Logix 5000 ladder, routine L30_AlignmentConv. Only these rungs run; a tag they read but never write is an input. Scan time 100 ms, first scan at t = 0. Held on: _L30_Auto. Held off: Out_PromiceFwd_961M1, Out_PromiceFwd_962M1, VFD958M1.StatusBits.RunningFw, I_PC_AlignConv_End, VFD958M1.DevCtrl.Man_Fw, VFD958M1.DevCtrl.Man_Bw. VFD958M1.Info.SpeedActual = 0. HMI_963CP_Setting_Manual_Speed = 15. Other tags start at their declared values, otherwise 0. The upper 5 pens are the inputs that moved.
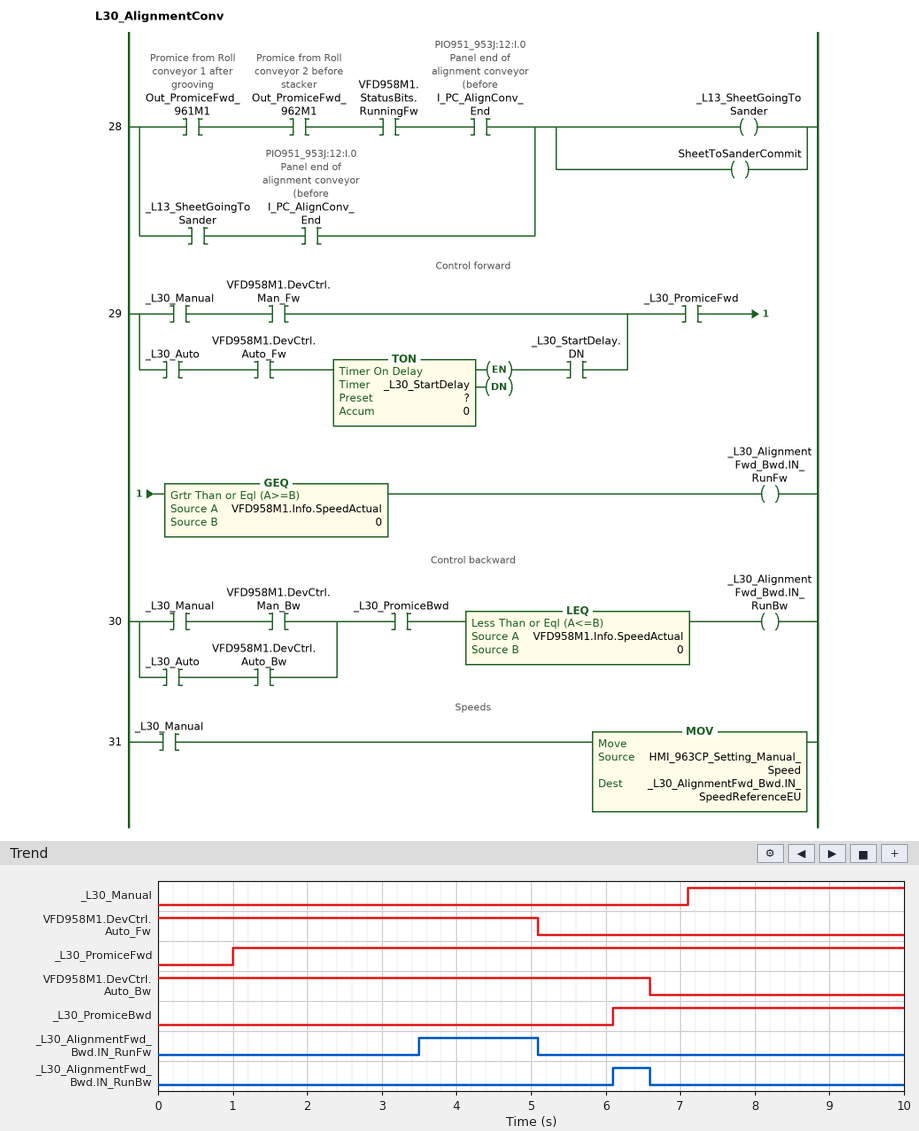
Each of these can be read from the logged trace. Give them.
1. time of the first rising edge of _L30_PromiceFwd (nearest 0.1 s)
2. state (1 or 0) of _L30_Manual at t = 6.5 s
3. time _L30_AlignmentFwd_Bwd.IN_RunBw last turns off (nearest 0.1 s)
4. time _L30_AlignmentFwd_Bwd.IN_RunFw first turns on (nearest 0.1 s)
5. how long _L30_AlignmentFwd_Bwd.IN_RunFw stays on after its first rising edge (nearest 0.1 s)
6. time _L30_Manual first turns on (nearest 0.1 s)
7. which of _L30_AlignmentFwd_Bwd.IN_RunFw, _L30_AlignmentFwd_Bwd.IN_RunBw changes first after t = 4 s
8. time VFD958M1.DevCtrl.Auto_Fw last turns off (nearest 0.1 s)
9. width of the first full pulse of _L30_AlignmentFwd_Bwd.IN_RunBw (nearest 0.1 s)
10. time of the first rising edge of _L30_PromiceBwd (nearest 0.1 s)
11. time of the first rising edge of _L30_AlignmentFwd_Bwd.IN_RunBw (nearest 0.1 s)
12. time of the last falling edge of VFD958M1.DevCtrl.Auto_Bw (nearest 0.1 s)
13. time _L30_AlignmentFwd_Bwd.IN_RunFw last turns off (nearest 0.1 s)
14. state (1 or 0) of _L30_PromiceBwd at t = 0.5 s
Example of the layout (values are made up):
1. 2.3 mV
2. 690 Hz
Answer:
1. 1.0 s
2. 0
3. 6.6 s
4. 3.5 s
5. 1.6 s
6. 7.1 s
7. _L30_AlignmentFwd_Bwd.IN_RunFw
8. 5.1 s
9. 0.5 s
10. 6.1 s
11. 6.1 s
12. 6.6 s
13. 5.1 s
14. 0
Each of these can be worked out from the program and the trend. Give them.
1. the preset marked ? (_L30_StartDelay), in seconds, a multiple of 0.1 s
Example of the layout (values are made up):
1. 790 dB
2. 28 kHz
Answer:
1. 3.5 s
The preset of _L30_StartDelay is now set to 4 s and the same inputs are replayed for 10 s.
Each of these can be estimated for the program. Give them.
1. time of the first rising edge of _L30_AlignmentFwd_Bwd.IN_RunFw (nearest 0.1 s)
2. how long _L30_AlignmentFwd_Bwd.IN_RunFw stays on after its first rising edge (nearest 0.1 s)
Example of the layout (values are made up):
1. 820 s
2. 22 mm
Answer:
1. 4.0 s
2. 1.1 s
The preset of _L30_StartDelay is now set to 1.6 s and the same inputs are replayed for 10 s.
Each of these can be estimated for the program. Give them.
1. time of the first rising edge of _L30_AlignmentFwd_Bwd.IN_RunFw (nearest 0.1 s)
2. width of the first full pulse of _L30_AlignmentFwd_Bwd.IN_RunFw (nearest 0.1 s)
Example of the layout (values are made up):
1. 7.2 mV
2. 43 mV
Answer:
1. 1.6 s
2. 3.5 s
